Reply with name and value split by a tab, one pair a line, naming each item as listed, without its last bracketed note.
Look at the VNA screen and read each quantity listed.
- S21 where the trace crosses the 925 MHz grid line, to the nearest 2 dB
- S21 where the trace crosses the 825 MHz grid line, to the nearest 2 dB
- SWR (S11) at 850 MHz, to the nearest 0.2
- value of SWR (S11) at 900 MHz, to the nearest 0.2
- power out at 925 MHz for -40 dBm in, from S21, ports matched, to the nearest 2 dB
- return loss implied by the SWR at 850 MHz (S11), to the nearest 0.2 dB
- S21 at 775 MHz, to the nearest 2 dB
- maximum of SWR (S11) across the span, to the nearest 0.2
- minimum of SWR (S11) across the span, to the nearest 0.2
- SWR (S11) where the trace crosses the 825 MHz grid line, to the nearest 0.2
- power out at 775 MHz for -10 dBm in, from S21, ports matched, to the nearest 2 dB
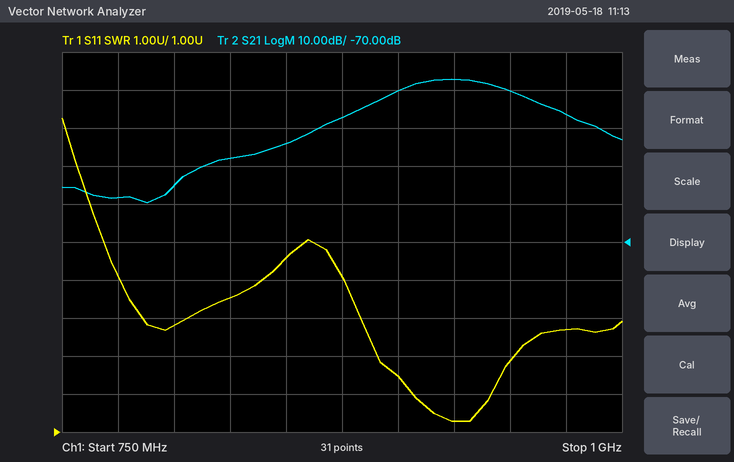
S21 where the trace crosses the 925 MHz grid line, to the nearest 2 dB	-28 dB
S21 where the trace crosses the 825 MHz grid line, to the nearest 2 dB	-48 dB
SWR (S11) at 850 MHz, to the nearest 0.2	5.6
value of SWR (S11) at 900 MHz, to the nearest 0.2	2.4
power out at 925 MHz for -40 dBm in, from S21, ports matched, to the nearest 2 dB	-68 dBm
return loss implied by the SWR at 850 MHz (S11), to the nearest 0.2 dB	3.2 dB
S21 at 775 MHz, to the nearest 2 dB	-58 dB
maximum of SWR (S11) across the span, to the nearest 0.2	9.2
minimum of SWR (S11) across the span, to the nearest 0.2	1.2
SWR (S11) where the trace crosses the 825 MHz grid line, to the nearest 0.2	4.6
power out at 775 MHz for -10 dBm in, from S21, ports matched, to the nearest 2 dB	-68 dBm
